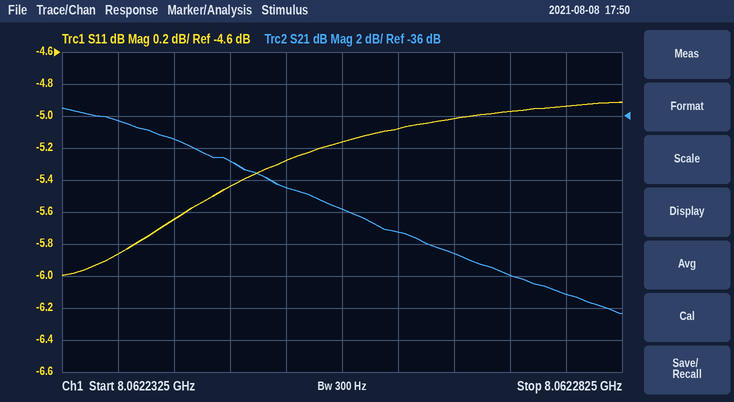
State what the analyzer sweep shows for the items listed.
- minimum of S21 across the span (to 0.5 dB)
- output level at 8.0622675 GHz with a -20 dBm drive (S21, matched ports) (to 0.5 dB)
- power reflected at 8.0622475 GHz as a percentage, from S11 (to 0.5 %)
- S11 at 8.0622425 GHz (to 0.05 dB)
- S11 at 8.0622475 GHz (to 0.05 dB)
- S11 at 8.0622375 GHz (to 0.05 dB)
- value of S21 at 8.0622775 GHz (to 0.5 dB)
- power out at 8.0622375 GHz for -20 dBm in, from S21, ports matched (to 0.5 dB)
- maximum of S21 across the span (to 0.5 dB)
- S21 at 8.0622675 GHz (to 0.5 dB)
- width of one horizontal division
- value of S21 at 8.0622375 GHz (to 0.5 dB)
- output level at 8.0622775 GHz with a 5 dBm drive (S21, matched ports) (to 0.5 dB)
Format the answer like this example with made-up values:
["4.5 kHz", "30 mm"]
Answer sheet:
["-48.5 dB", "-64.5 dBm", "28.5 %", "-5.65 dB", "-5.45 dB", "-5.85 dB", "-47.0 dB", "-56.5 dBm", "-35.5 dB", "-44.5 dB", "5 kHz", "-36.5 dB", "-42.0 dBm"]
